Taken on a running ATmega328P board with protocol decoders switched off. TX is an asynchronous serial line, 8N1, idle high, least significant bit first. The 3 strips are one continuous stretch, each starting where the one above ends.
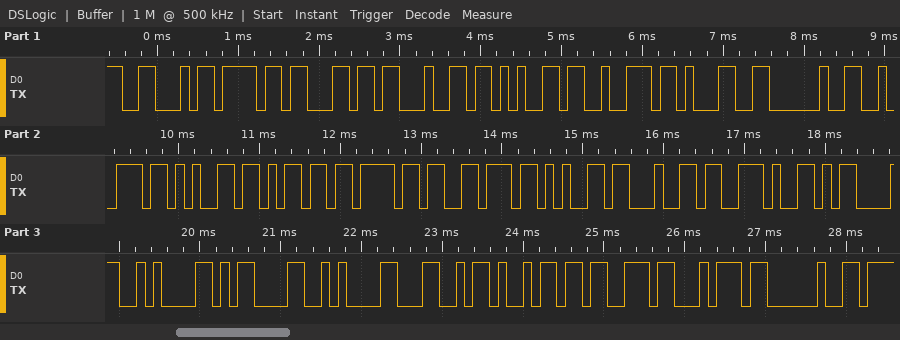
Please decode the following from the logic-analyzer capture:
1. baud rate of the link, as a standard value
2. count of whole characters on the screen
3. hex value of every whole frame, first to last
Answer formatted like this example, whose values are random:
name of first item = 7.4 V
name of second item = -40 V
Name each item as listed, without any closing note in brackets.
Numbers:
baud rate of the link, as a standard value = 9600 baud
count of whole characters on the screen = 25
hex value of every whole frame, first to last = 46 6F 6C 64 65 72 31 20 72 65 6D 6F 76 65 64 2E 0D 0A 0D 0A 4C 69 73 74 20
